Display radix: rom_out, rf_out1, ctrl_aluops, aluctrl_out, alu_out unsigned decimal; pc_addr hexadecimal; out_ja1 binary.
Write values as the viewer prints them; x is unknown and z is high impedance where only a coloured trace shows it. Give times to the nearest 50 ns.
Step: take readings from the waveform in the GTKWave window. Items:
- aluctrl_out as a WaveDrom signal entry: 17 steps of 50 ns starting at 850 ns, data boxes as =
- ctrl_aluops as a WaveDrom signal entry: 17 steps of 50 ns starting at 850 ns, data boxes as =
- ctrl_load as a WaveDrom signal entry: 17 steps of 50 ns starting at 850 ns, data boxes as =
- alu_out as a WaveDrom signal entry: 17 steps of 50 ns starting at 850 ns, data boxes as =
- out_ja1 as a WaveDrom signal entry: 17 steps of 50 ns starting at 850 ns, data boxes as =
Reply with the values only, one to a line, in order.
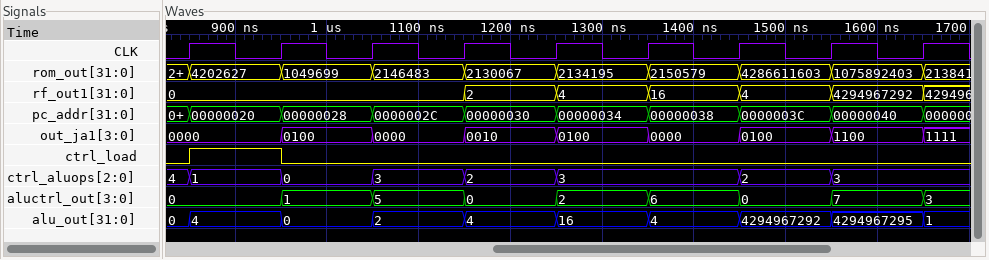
{name: 'aluctrl_out', wave: '=.=.=.=.=.=.=.=.=', data: '0 1 5 0 2 6 0 7 3'}
{name: 'ctrl_aluops', wave: '=.=.=.=.=...=.=..', data: '1 0 3 2 3 2 3'}
{name: 'ctrl_load', wave: '1.0..............'}
{name: 'alu_out', wave: '=.=.=.=.=.=.=.=.=', data: '4 0 2 4 16 4 4294967292 4294967295 1'}
{name: 'out_ja1', wave: '=.=.=.=.=.=.=.=.=', data: '0000 0100 0000 0010 0100 0000 0100 1100 1111'}
